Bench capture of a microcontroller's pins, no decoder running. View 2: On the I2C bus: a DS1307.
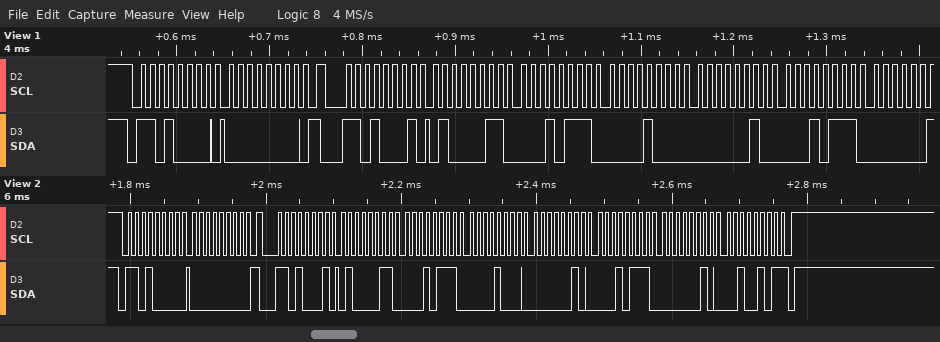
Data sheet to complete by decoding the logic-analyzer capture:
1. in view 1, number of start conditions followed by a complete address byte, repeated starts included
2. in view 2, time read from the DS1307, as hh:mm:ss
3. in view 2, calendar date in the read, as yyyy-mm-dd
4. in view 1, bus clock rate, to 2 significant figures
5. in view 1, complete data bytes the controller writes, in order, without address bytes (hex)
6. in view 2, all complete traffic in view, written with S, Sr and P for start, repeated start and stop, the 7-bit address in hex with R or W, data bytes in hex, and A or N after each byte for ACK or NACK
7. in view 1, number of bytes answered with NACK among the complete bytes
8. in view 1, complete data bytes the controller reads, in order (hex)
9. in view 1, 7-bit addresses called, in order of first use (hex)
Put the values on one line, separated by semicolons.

2; 08:17:43; 2025-02-17; 100 kHz; 00; S 68W A 00 A Sr 68R A 43 A 17 A 08 A 02 A 17 A 02 A 25 N P; 0; 43 17 08 02 17; 0x68
